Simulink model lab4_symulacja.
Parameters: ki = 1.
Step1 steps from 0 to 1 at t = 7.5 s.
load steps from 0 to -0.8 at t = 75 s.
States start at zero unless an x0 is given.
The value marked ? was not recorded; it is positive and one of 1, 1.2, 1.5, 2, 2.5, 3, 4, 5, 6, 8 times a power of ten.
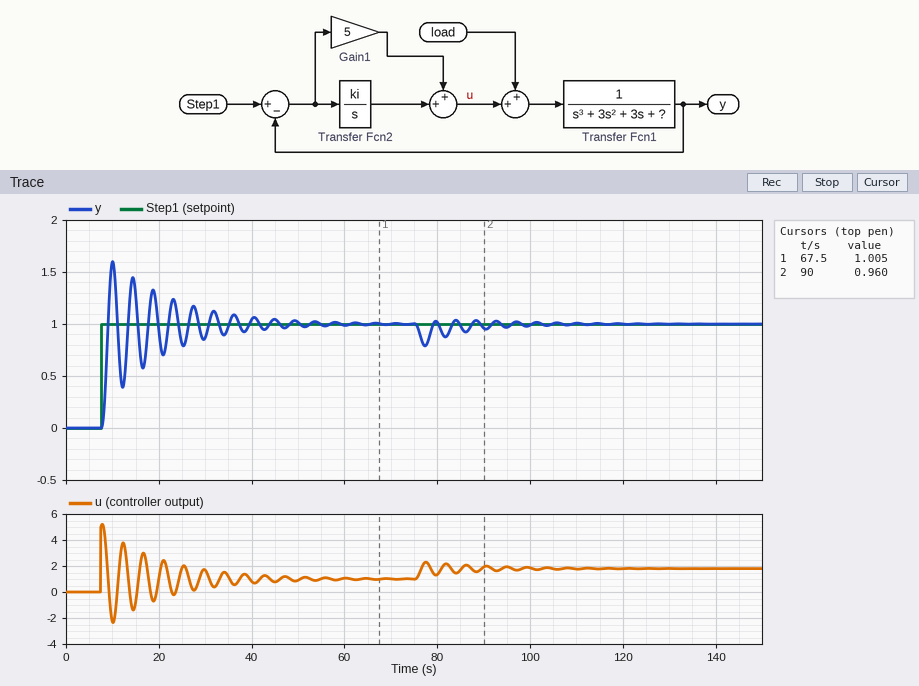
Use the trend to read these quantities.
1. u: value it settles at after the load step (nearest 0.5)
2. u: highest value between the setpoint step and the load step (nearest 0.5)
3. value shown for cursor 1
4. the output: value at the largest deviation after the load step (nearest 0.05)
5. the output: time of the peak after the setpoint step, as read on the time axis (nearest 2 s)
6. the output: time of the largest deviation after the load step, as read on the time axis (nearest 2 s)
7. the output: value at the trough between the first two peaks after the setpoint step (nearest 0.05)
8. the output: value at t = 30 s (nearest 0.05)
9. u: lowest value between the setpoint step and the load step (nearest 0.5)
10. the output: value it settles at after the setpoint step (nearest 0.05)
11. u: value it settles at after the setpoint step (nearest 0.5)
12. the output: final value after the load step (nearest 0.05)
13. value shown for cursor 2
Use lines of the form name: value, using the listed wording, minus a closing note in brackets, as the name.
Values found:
u: value it settles at after the load step: 2.0
u: highest value between the setpoint step and the load step: 5.0
value shown for cursor 1: 1.005
the output: value at the largest deviation after the load step: 0.80
the output: time of the peak after the setpoint step, as read on the time axis: 10 s
the output: time of the largest deviation after the load step, as read on the time axis: 78 s
the output: value at the trough between the first two peaks after the setpoint step: 0.40
the output: value at t = 30 s: 0.85
u: lowest value between the setpoint step and the load step: -2.5
the output: value it settles at after the setpoint step: 1.00
u: value it settles at after the setpoint step: 1.0
the output: final value after the load step: 1.00
value shown for cursor 2: 0.960
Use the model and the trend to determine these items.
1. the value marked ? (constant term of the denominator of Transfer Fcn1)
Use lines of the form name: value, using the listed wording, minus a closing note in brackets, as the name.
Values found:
the value marked ?: 1
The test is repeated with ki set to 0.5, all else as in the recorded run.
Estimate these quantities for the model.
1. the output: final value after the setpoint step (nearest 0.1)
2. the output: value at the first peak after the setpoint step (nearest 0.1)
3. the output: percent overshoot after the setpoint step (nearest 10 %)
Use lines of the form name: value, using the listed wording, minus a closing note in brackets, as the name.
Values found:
the output: final value after the setpoint step: 1.0
the output: value at the first peak after the setpoint step: 1.5
the output: percent overshoot after the setpoint step: 50 %
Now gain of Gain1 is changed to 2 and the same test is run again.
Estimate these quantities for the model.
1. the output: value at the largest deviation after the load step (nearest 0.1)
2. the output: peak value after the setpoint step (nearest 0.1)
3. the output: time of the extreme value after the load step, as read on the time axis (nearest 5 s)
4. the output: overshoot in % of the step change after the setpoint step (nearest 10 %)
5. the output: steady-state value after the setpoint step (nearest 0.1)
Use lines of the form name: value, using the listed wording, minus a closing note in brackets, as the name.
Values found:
the output: value at the largest deviation after the load step: 0.7
the output: peak value after the setpoint step: 1.4
the output: time of the extreme value after the load step, as read on the time axis: 80 s
the output: overshoot in % of the step change after the setpoint step: 40 %
the output: steady-state value after the setpoint step: 1.0
